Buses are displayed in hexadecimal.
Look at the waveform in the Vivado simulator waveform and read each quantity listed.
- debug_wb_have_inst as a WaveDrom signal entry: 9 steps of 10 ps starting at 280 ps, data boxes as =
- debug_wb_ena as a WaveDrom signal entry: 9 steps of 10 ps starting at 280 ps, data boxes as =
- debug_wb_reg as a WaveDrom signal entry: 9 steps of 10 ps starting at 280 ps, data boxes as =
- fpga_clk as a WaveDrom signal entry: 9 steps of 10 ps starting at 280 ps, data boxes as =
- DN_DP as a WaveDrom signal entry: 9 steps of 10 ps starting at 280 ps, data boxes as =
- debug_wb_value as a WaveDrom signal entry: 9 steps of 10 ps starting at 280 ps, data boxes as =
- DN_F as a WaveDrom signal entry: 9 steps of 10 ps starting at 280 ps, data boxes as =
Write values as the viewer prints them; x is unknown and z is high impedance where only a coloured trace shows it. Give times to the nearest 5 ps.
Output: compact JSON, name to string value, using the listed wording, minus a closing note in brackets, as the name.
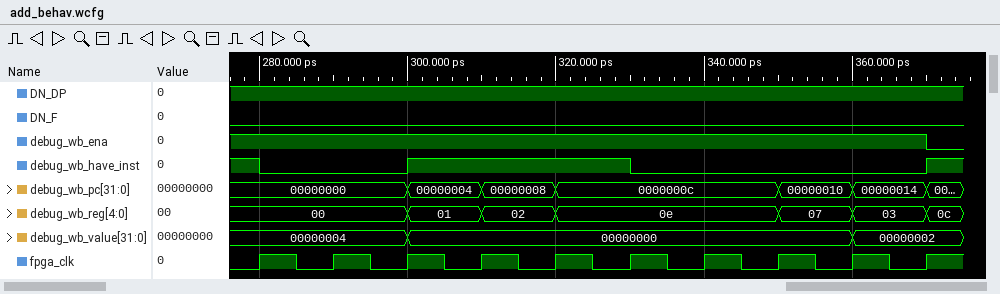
{"debug_wb_have_inst as a WaveDrom signal entry: 9 steps of 10 ps starting at 280 ps, data boxes as =": "{name: 'debug_wb_have_inst', wave: '0.1..0...'}", "debug_wb_ena as a WaveDrom signal entry: 9 steps of 10 ps starting at 280 ps, data boxes as =": "{name: 'debug_wb_ena', wave: '1........'}", "debug_wb_reg as a WaveDrom signal entry: 9 steps of 10 ps starting at 280 ps, data boxes as =": "{name: 'debug_wb_reg', wave: '=.===..==', data: '00 01 02 0e 07 03'}", "fpga_clk as a WaveDrom signal entry: 9 steps of 10 ps starting at 280 ps, data boxes as =": "{name: 'fpga_clk', wave: 'p........'}", "DN_DP as a WaveDrom signal entry: 9 steps of 10 ps starting at 280 ps, data boxes as =": "{name: 'DN_DP', wave: '1........'}", "debug_wb_value as a WaveDrom signal entry: 9 steps of 10 ps starting at 280 ps, data boxes as =": "{name: 'debug_wb_value', wave: '=.=.....=', data: '00000004 00000000 00000002'}", "DN_F as a WaveDrom signal entry: 9 steps of 10 ps starting at 280 ps, data boxes as =": "{name: 'DN_F', wave: '0........'}"}
